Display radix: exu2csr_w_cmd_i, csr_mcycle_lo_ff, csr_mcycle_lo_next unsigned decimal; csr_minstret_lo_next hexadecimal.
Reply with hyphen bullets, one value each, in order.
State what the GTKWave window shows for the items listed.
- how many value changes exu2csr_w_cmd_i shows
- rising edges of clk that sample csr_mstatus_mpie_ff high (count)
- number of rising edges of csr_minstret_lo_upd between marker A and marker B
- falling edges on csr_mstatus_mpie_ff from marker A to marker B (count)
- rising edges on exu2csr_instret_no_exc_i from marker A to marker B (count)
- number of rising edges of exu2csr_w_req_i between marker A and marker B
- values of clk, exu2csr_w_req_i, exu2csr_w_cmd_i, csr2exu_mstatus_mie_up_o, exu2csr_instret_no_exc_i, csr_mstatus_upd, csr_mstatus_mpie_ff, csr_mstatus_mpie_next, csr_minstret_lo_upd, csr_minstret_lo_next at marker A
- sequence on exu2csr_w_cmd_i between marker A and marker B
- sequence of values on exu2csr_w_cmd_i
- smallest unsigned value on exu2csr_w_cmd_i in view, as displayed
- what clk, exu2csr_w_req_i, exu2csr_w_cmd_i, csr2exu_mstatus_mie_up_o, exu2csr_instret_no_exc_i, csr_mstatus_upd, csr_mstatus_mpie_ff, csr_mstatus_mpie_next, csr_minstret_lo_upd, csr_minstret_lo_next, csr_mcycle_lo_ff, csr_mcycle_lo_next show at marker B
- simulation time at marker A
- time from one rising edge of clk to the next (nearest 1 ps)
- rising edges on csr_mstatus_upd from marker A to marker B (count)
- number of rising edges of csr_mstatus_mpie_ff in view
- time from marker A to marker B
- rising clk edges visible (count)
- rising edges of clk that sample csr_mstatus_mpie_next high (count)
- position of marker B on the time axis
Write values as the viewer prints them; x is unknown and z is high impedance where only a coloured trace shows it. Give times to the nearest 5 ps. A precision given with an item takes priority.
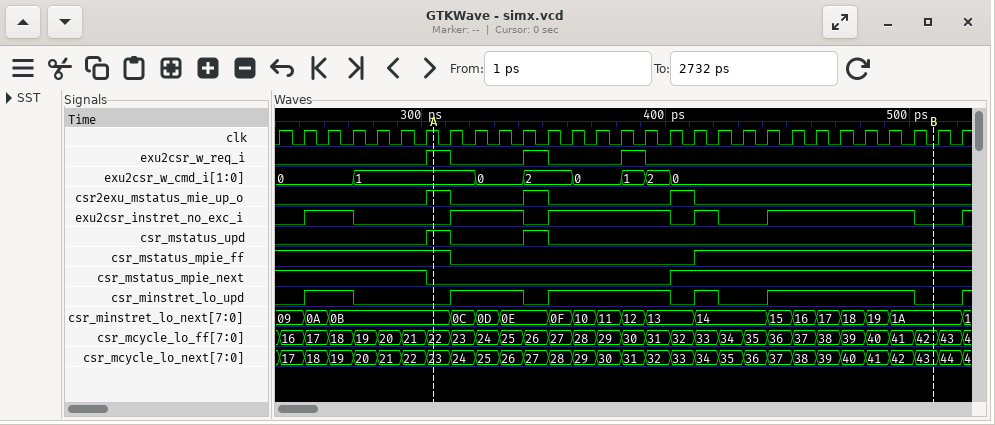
- 7
- 19
- 4
- 1
- 4
- 2
- clk=1, exu2csr_w_req_i=1, exu2csr_w_cmd_i=1, csr2exu_mstatus_mie_up_o=1, exu2csr_instret_no_exc_i=0, csr_mstatus_upd=1, csr_mstatus_mpie_ff=1, csr_mstatus_mpie_next=0, csr_minstret_lo_upd=0, csr_minstret_lo_next=0B
- 1, 0, 2, 0, 1, 2, 0
- 0, 1, 0, 2, 0, 1, 2, 0
- 0
- clk=0, exu2csr_w_req_i=0, exu2csr_w_cmd_i=0, csr2exu_mstatus_mie_up_o=0, exu2csr_instret_no_exc_i=0, csr_mstatus_upd=0, csr_mstatus_mpie_ff=1, csr_mstatus_mpie_next=1, csr_minstret_lo_upd=0, csr_minstret_lo_next=1A, csr_mcycle_lo_ff=42, csr_mcycle_lo_next=43
- 305 ps
- 10 ps
- 1
- 1
- 205 ps
- 29
- 19
- 510 ps
